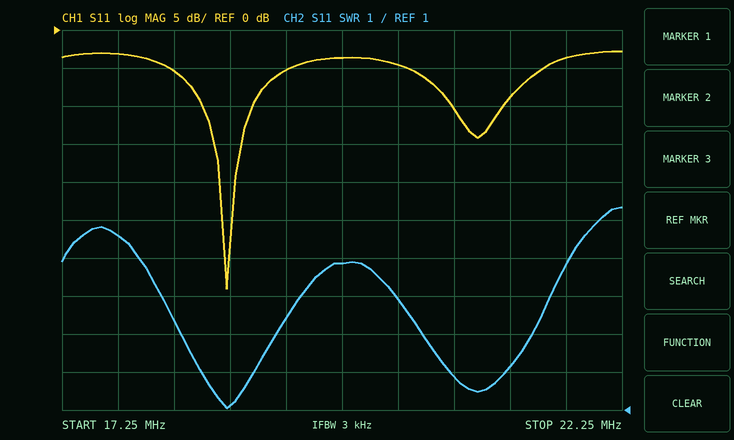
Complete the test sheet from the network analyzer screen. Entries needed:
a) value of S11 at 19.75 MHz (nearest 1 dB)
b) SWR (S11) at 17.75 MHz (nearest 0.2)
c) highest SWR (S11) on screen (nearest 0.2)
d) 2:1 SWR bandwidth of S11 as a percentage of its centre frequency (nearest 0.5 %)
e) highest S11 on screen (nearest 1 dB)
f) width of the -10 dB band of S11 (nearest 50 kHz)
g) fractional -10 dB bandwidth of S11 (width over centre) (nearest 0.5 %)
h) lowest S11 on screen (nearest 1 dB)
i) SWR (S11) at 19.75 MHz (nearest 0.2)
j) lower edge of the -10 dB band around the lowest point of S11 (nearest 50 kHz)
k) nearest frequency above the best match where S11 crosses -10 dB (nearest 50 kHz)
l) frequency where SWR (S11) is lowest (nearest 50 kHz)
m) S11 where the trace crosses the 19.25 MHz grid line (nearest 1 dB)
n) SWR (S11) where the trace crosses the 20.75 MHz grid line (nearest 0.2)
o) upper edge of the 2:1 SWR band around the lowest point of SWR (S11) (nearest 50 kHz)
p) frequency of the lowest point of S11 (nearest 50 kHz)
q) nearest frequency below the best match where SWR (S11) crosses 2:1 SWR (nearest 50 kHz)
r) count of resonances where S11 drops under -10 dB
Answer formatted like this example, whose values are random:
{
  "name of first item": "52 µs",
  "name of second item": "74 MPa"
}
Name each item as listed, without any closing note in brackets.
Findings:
{
  "value of S11 at 19.75 MHz": "-4 dB",
  "SWR (S11) at 17.75 MHz": "5.6",
  "highest SWR (S11) on screen": "6.4",
  "2:1 SWR bandwidth of S11 as a percentage of its centre frequency": "2.5 %",
  "highest S11 on screen": "-3 dB",
  "width of the -10 dB band of S11": "450 kHz",
  "fractional -10 dB bandwidth of S11 (width over centre)": "2.5 %",
  "lowest S11 on screen": "-34 dB",
  "SWR (S11) at 19.75 MHz": "4.8",
  "lower edge of the -10 dB band around the lowest point of S11": "18.50 MHz",
  "nearest frequency above the best match where S11 crosses -10 dB": "18.95 MHz",
  "frequency where SWR (S11) is lowest": "18.70 MHz",
  "S11 where the trace crosses the 19.25 MHz grid line": "-5 dB",
  "SWR (S11) where the trace crosses the 20.75 MHz grid line": "1.8",
  "upper edge of the 2:1 SWR band around the lowest point of SWR (S11)": "18.95 MHz",
  "frequency of the lowest point of S11": "18.70 MHz",
  "nearest frequency below the best match where SWR (S11) crosses 2:1 SWR": "18.50 MHz",
  "count of resonances where S11 drops under -10 dB": "2"
}
